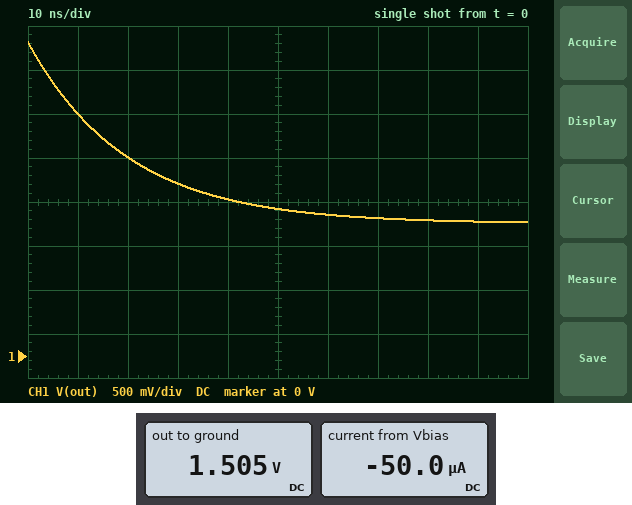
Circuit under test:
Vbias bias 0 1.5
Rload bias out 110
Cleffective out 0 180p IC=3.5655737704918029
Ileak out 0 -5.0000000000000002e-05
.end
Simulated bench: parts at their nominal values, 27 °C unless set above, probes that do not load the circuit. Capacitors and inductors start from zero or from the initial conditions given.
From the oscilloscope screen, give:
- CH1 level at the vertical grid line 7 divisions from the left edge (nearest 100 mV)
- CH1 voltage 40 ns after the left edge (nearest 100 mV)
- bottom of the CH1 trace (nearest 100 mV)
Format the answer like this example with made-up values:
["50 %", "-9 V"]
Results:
["1.6 V", "1.8 V", "1.5 V"]
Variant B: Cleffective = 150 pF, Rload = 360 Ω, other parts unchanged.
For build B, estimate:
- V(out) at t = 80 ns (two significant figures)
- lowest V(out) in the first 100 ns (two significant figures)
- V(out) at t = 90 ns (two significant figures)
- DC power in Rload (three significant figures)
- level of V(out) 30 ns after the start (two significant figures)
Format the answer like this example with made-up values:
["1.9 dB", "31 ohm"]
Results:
["2.0 V", "1.8 V", "1.9 V", "900 nW", "2.7 V"]
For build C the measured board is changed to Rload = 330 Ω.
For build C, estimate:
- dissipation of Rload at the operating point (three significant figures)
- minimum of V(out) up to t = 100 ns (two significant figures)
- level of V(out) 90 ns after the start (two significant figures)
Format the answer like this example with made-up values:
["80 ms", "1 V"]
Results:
["825 nW", "1.9 V", "2.0 V"]
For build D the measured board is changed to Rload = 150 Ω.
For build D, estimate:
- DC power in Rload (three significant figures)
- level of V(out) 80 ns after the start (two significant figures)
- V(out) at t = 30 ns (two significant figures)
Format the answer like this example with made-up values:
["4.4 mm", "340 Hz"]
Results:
["375 nW", "1.6 V", "2.2 V"]
